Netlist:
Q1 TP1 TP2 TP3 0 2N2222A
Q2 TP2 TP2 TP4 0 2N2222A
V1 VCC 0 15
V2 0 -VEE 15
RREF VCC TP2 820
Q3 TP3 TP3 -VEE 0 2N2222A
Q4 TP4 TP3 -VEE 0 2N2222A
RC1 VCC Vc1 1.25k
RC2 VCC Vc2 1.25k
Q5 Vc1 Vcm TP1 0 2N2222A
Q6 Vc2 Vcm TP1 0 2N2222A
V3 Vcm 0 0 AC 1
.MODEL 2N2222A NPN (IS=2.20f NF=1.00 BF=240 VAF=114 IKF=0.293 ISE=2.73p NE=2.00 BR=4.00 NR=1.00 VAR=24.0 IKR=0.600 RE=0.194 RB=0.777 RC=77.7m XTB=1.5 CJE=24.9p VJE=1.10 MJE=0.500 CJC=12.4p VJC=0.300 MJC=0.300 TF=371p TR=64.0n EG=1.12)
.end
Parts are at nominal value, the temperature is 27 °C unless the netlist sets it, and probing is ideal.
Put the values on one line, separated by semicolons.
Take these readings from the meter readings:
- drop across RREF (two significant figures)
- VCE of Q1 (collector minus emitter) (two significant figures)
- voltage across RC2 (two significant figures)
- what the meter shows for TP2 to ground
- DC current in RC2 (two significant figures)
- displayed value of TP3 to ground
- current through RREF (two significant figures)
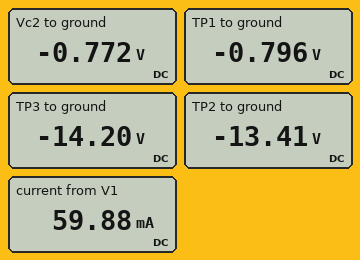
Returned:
28 V; 13 V; 16 V; -13.41 V; 13 mA; -14.20 V; 35 mA
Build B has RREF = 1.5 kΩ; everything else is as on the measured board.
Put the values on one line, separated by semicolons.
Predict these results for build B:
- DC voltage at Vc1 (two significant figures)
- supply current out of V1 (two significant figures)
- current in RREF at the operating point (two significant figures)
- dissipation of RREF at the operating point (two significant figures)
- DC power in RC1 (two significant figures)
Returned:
3.2 V; 38 mA; 19 mA; 540 mW; 110 mW
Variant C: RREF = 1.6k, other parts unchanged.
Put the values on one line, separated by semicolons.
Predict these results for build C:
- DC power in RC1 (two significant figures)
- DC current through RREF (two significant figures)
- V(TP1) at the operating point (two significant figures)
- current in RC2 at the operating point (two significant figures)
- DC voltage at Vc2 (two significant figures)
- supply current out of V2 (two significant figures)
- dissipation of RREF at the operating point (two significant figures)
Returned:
98 mW; 18 mA; -750 mV; 8.9 mA; 3.9 V; 36 mA; 510 mW
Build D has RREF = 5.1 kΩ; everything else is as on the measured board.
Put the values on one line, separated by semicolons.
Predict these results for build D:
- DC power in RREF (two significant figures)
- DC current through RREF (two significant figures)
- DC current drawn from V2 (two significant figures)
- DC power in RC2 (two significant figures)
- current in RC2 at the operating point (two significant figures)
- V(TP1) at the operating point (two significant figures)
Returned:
160 mW; 5.6 mA; 11 mA; 9.7 mW; 2.8 mA; -720 mV
